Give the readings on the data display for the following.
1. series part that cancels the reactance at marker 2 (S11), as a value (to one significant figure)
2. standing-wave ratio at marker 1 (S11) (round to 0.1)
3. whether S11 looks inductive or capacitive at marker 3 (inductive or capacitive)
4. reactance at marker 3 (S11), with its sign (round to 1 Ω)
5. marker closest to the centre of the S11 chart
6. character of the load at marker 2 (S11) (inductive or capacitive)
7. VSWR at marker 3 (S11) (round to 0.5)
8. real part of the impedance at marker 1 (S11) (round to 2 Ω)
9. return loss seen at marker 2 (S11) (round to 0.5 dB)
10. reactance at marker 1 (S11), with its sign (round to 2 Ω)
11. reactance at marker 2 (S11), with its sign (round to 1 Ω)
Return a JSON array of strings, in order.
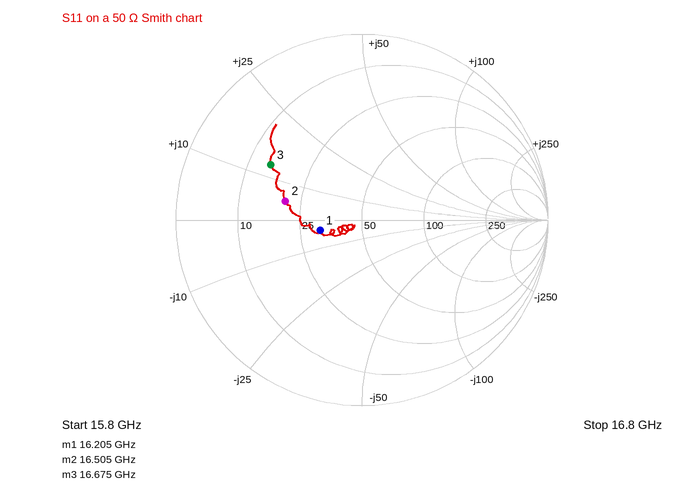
["2 pF", "1.6", "inductive", "+13 Ω", "marker 1", "inductive", "3.5", "32 Ω", "7.5 dB", "-4 Ω", "+5 Ω"]
